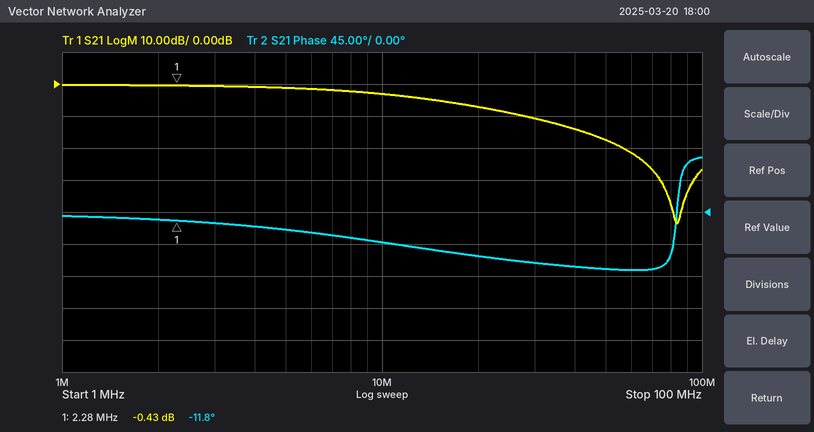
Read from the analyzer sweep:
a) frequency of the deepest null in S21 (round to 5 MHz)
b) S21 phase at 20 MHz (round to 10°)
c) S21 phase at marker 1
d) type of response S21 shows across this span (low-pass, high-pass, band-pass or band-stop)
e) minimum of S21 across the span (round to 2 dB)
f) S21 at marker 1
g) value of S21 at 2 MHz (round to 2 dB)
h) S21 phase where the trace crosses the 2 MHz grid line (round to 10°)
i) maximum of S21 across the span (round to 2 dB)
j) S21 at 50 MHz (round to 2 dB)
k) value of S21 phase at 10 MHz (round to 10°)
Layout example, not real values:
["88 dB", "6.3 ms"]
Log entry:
["85 MHz", "-60°", "-11.8°", "low-pass", "-44 dB", "-0.43 dB", "0 dB", "-10°", "0 dB", "-18 dB", "-40°"]
